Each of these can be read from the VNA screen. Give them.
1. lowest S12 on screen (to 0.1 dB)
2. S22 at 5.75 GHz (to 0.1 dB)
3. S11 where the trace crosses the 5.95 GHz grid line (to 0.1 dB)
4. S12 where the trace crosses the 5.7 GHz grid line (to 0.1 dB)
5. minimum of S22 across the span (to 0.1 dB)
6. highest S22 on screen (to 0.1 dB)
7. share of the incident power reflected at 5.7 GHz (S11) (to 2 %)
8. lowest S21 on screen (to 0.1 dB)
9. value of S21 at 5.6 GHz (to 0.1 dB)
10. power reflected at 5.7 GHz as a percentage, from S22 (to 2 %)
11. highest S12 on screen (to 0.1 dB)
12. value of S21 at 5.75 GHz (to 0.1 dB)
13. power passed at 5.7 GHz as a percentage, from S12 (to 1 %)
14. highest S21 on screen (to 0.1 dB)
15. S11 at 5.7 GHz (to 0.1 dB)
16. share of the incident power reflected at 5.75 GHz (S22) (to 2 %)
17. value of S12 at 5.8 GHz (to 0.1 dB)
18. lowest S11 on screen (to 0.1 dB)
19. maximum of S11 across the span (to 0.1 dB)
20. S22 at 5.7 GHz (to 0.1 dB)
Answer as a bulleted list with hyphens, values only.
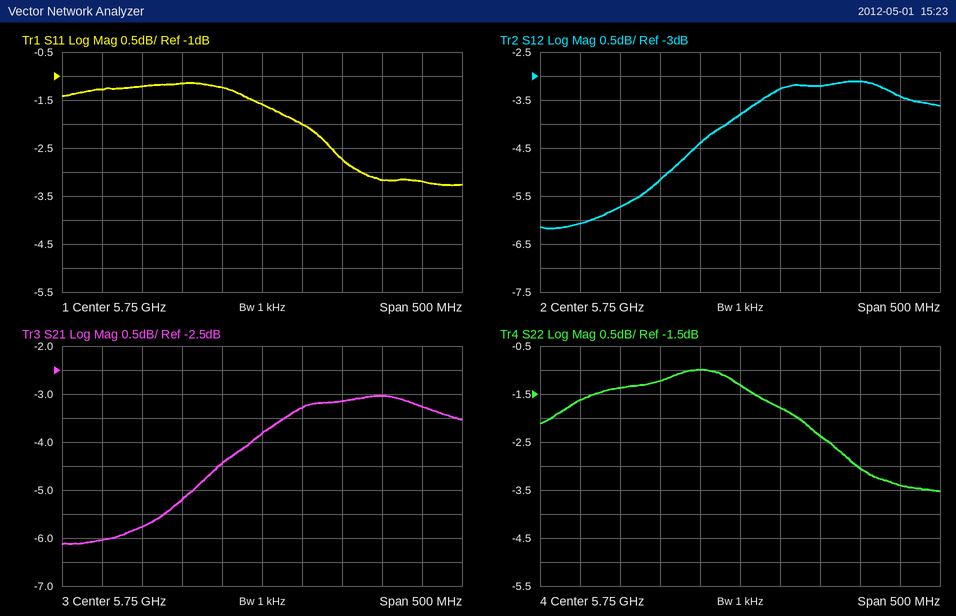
- -6.2 dB
- -1.3 dB
- -3.2 dB
- -4.4 dB
- -3.5 dB
- -1.0 dB
- 76 %
- -6.1 dB
- -5.8 dB
- 80 %
- -3.1 dB
- -3.8 dB
- 36 %
- -3.0 dB
- -1.2 dB
- 74 %
- -3.3 dB
- -3.3 dB
- -1.1 dB
- -1.0 dB
